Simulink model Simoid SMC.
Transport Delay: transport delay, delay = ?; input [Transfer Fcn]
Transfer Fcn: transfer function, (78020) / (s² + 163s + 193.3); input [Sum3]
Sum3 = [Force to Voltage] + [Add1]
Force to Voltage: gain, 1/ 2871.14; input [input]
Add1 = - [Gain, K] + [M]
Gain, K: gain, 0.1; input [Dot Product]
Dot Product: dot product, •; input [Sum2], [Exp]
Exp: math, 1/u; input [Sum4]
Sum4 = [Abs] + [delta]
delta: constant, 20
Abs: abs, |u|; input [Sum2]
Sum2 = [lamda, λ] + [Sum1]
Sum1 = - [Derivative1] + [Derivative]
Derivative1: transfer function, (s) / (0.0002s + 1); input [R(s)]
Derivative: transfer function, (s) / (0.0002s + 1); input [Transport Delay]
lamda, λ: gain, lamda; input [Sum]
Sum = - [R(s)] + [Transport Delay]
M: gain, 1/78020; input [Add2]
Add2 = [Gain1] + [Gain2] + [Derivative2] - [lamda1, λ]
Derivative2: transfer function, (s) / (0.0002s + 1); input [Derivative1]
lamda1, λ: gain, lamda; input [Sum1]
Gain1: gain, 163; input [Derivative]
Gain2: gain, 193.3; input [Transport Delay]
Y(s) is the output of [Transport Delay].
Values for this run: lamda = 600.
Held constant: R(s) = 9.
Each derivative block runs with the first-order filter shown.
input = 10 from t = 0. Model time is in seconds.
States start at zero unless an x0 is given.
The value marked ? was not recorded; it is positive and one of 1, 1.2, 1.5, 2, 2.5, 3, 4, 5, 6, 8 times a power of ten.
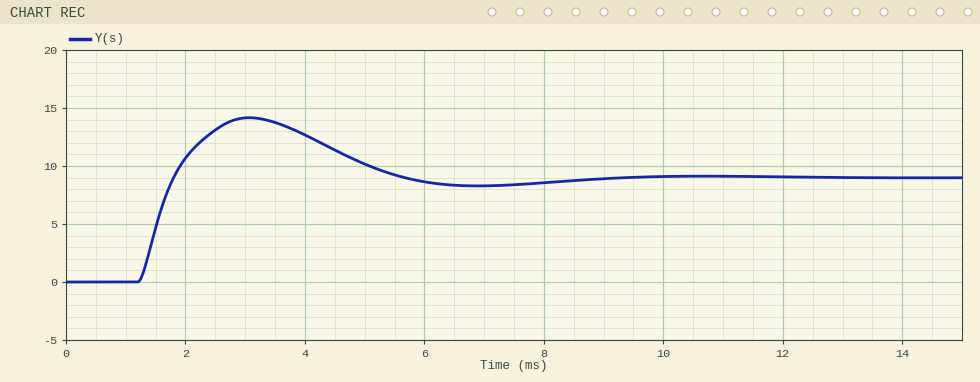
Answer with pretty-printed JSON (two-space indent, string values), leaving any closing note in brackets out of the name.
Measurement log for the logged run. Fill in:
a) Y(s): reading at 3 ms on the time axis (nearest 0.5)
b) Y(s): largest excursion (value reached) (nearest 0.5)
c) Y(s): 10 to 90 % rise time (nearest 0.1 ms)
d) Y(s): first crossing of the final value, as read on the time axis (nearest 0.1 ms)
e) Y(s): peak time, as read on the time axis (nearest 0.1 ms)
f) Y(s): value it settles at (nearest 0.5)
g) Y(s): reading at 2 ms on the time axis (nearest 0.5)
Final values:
{
  "Y(s): reading at 3 ms on the time axis": "14.0",
  "Y(s): largest excursion (value reached)": "14.0",
  "Y(s): 10 to 90 % rise time": "0.4 ms",
  "Y(s): first crossing of the final value, as read on the time axis": "1.8 ms",
  "Y(s): peak time, as read on the time axis": "3.1 ms",
  "Y(s): value it settles at": "9.0",
  "Y(s): reading at 2 ms on the time axis": "10.5"
}
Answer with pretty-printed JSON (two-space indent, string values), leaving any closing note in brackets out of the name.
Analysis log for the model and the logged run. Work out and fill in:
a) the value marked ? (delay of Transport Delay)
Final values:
{
  "the value marked ?": "0.0012"
}
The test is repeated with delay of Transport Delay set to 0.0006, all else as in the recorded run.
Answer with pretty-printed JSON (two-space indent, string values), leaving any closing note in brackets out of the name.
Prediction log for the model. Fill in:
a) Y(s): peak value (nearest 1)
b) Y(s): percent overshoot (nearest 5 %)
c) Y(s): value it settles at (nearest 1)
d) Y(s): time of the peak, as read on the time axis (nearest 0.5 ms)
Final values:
{
  "Y(s): peak value": "12",
  "Y(s): percent overshoot": "35 %",
  "Y(s): value it settles at": "9",
  "Y(s): time of the peak, as read on the time axis": "2.0 ms"
}
